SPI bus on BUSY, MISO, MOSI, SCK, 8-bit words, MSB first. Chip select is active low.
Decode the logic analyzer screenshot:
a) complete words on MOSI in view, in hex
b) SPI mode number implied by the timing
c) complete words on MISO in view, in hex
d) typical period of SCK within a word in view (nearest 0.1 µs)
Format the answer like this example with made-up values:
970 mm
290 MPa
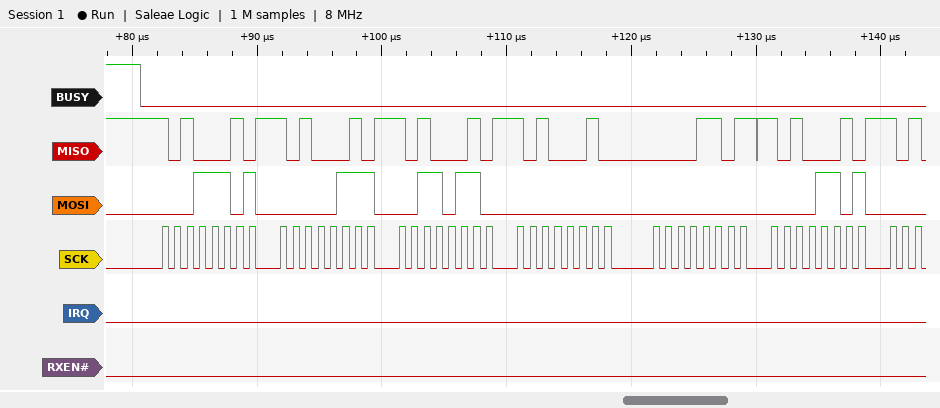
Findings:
1D, 07, 36, 00, 00, 0D
0
A2, A2, A2, A2, 0D, A2
1 µs
